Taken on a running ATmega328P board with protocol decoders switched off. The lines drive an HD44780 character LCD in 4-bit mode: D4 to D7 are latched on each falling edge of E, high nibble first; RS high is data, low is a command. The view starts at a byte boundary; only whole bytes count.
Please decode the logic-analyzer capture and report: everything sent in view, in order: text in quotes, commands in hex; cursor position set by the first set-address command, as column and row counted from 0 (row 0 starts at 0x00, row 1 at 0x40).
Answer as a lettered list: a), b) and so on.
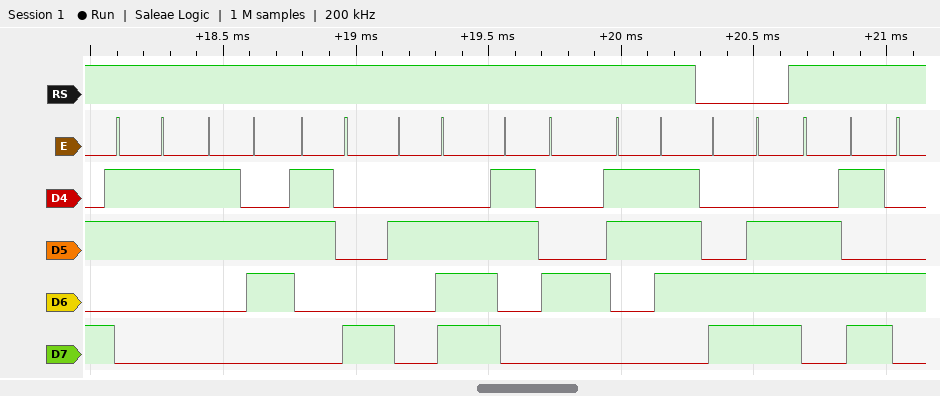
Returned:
a) "368.47" 0xCE "m"
b) column 14, row 1
